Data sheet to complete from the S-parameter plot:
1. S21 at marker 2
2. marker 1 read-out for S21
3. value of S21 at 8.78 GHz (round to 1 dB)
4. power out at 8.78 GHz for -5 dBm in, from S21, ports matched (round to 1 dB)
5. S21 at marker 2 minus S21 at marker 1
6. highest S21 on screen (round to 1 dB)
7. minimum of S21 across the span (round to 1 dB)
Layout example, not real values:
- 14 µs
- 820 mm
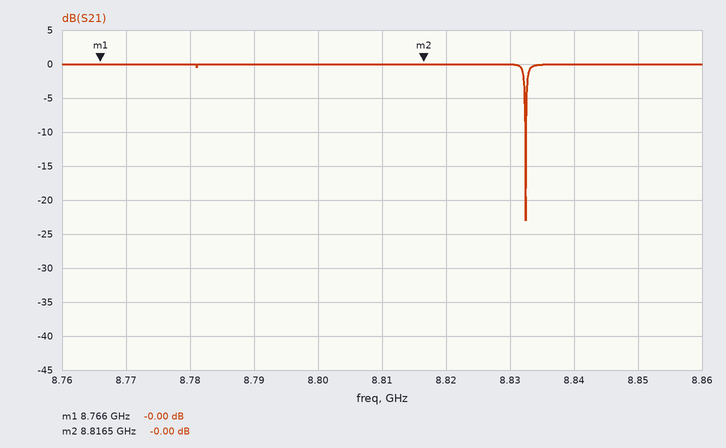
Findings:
- -0.00 dB
- -0.00 dB
- 0 dB
- -5 dBm
- 0.00 dB
- 0 dB
- -23 dB
